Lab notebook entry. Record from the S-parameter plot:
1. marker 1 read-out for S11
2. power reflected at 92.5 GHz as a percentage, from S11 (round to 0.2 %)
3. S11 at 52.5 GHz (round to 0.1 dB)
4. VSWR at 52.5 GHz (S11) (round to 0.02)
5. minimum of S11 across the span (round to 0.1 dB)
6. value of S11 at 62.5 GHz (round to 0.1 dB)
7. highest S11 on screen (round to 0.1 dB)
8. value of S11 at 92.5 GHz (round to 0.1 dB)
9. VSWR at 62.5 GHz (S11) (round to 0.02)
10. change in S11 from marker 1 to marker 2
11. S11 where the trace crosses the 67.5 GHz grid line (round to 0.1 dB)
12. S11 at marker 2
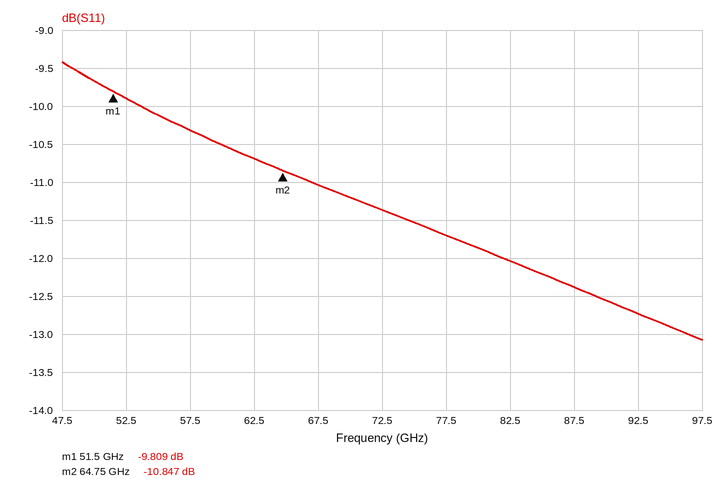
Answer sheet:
-9.809 dB
5.4 %
-9.9 dB
1.94
-13.1 dB
-10.7 dB
-9.4 dB
-12.7 dB
1.82
-1.038 dB
-11.0 dB
-10.847 dB
